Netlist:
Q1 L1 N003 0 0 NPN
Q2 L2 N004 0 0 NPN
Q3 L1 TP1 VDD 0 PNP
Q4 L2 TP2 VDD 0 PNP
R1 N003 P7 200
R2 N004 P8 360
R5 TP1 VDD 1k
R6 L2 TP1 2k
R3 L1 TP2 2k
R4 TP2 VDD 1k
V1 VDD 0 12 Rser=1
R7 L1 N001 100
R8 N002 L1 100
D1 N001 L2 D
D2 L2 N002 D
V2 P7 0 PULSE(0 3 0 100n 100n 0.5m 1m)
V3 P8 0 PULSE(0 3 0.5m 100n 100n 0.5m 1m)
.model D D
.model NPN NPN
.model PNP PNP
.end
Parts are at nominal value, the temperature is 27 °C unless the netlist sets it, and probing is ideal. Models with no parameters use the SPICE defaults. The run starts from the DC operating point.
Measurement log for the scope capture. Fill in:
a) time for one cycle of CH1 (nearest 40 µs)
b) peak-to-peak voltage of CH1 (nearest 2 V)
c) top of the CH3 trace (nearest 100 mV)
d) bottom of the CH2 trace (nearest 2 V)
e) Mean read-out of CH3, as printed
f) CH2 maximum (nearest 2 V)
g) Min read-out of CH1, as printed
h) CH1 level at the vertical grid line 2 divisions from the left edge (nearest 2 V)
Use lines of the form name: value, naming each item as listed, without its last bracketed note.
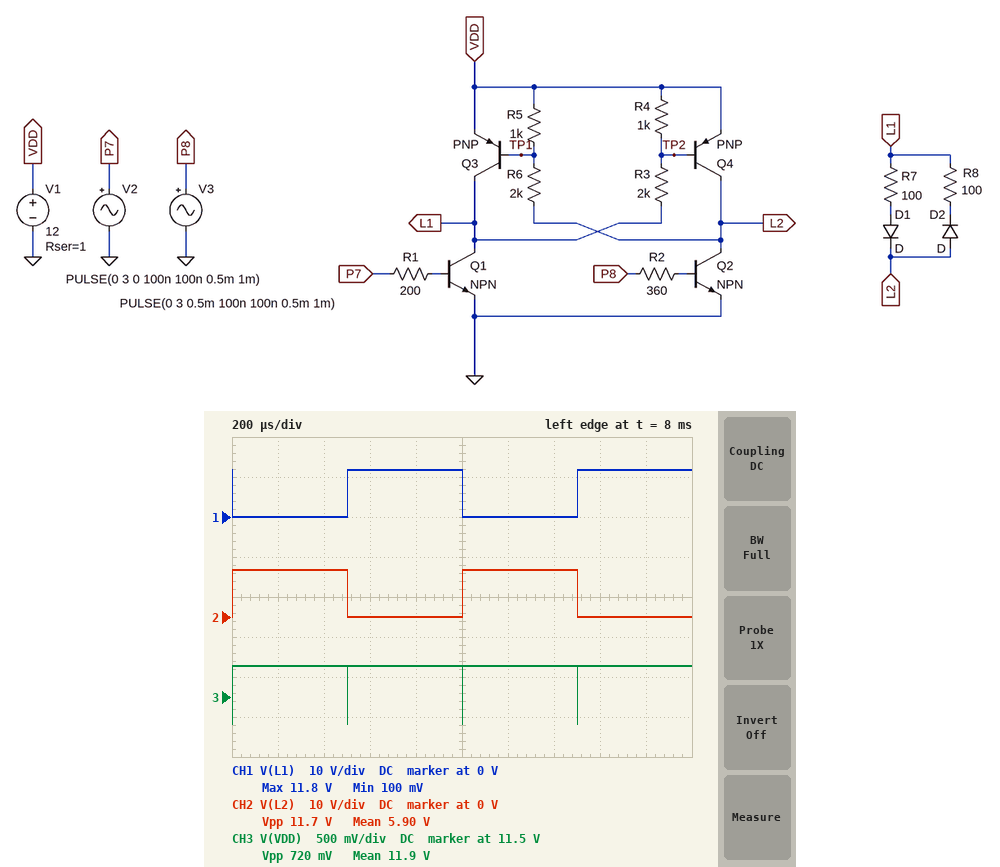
time for one cycle of CH1: 1.00 ms
peak-to-peak voltage of CH1: 12 V
top of the CH3 trace: 11.9 V
bottom of the CH2 trace: 0 V
Mean read-out of CH3, as printed: 11.9 V
CH2 maximum: 12 V
Min read-out of CH1, as printed: 100 mV
CH1 level at the vertical grid line 2 divisions from the left edge: 0 V
